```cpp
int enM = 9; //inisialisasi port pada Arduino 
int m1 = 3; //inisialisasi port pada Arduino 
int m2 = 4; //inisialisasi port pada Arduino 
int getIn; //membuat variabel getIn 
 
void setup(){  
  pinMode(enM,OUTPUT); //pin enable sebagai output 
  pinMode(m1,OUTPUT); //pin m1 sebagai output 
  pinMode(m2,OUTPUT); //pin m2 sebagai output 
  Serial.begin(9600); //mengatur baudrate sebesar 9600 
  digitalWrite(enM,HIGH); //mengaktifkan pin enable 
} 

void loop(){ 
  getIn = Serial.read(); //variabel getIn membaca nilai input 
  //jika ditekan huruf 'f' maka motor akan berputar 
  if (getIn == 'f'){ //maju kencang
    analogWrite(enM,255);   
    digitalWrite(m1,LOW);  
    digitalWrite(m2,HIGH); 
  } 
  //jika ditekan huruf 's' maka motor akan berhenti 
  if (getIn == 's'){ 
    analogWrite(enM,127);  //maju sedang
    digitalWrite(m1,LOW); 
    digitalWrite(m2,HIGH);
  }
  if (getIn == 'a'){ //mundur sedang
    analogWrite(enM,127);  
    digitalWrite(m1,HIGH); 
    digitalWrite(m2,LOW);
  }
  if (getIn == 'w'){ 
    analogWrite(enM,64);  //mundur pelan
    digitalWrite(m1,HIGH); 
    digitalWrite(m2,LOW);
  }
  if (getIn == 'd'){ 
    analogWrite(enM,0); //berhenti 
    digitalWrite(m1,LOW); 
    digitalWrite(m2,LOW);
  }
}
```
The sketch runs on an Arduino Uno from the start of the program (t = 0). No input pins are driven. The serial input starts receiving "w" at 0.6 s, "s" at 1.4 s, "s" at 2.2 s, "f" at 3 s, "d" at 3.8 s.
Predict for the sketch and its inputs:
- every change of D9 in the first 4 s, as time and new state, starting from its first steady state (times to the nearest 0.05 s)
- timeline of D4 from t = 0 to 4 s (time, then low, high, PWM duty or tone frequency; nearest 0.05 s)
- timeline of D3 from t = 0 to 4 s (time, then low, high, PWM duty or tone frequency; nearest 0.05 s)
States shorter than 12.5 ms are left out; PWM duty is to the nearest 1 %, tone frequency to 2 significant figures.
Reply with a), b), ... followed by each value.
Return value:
a) 0 s high; 0.6 s PWM 25 %; 1.4 s PWM 50 %; 3 s high; 3.8 s low
b) 0 s low; 1.4 s high; 3.8 s low
c) 0 s low; 0.6 s high; 1.4 s low
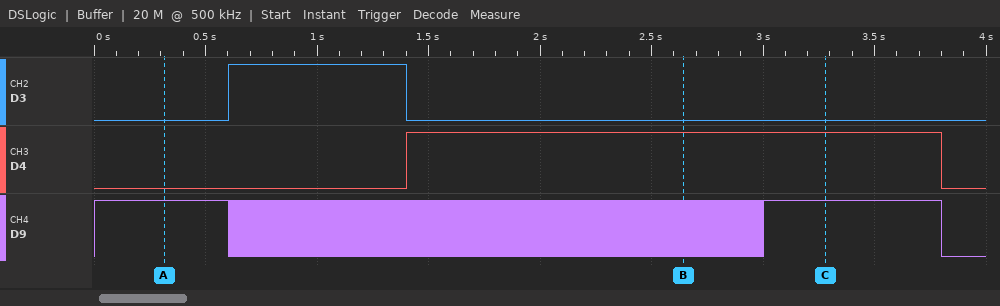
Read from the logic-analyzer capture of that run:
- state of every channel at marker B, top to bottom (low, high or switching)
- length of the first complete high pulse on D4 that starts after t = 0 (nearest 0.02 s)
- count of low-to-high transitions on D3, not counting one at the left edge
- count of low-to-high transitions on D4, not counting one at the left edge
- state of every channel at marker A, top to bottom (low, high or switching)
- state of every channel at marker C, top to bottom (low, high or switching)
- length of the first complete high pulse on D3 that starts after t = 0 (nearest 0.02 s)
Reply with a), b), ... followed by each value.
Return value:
a) D3 low, D4 high, D9 switching
b) 2.40 s
c) 1
d) 1
e) D3 low, D4 low, D9 high
f) D3 low, D4 high, D9 high
g) 0.80 s
